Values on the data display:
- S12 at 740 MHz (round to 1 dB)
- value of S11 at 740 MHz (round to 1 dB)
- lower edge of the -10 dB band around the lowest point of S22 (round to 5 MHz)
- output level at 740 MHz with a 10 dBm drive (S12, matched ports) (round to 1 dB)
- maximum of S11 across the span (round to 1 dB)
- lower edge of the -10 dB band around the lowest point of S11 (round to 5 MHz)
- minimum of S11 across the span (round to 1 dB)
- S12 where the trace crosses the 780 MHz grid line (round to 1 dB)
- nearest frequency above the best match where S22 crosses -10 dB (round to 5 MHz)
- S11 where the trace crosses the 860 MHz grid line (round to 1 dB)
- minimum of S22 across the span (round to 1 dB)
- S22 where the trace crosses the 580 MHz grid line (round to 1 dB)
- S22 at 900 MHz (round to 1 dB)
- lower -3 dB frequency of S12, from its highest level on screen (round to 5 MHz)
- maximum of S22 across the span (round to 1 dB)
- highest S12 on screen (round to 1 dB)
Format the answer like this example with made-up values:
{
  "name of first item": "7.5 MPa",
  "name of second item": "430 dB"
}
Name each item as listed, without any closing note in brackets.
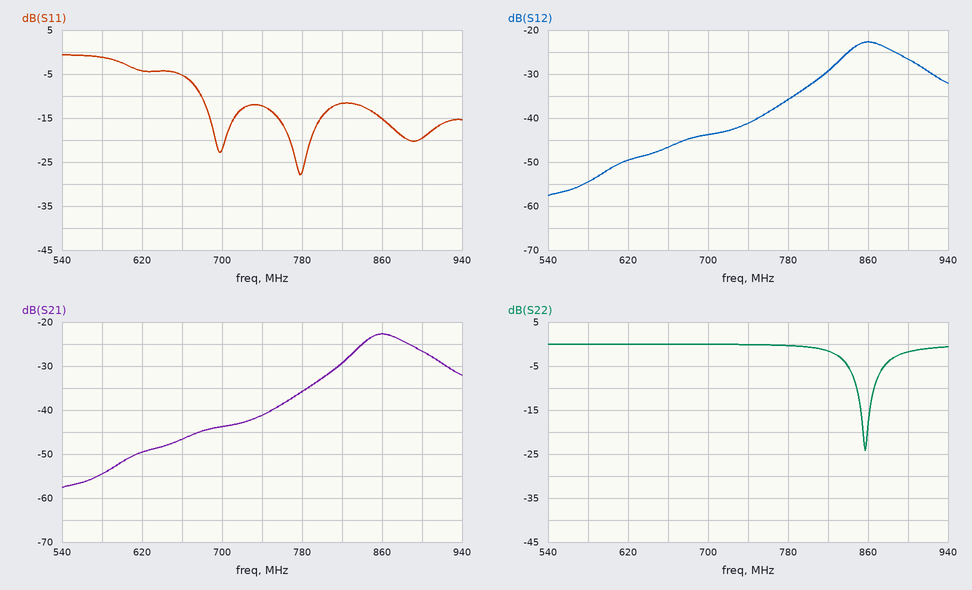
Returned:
{
  "S12 at 740 MHz": "-41 dB",
  "value of S11 at 740 MHz": "-12 dB",
  "lower edge of the -10 dB band around the lowest point of S22": "850 MHz",
  "output level at 740 MHz with a 10 dBm drive (S12, matched ports)": "-31 dBm",
  "maximum of S11 across the span": "-1 dB",
  "lower edge of the -10 dB band around the lowest point of S11": "680 MHz",
  "minimum of S11 across the span": "-28 dB",
  "S12 where the trace crosses the 780 MHz grid line": "-36 dB",
  "nearest frequency above the best match where S22 crosses -10 dB": "865 MHz",
  "S11 where the trace crosses the 860 MHz grid line": "-15 dB",
  "minimum of S22 across the span": "-24 dB",
  "S22 where the trace crosses the 580 MHz grid line": "0 dB",
  "S22 at 900 MHz": "-2 dB",
  "lower -3 dB frequency of S12, from its highest level on screen": "835 MHz",
  "maximum of S22 across the span": "0 dB",
  "highest S12 on screen": "-23 dB"
}
